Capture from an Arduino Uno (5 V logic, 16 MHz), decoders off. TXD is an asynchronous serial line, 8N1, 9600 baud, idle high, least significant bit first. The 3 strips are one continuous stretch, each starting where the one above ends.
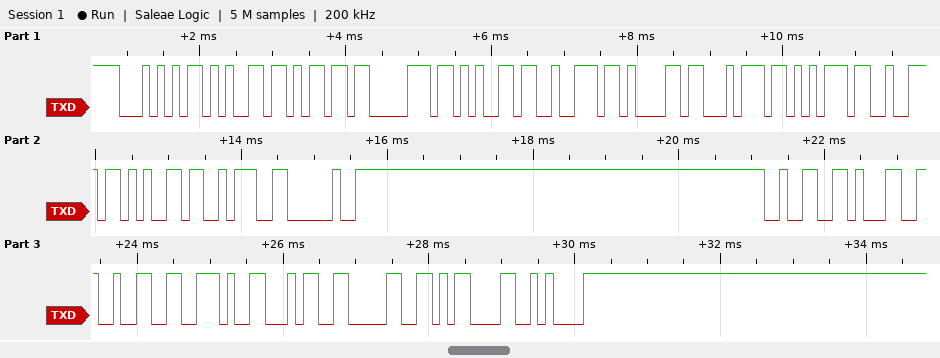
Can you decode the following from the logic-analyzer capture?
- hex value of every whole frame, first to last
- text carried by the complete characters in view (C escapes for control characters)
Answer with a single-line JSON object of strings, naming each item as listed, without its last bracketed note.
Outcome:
{"hex value of every whole frame, first to last": "54 65 6D 70 65 72 61 74 75 72 65 3A 20 32 31 32 2E 34 30 0D 0A", "text carried by the complete characters in view": "\"Temperature: 212.40\\r\\n\""}
